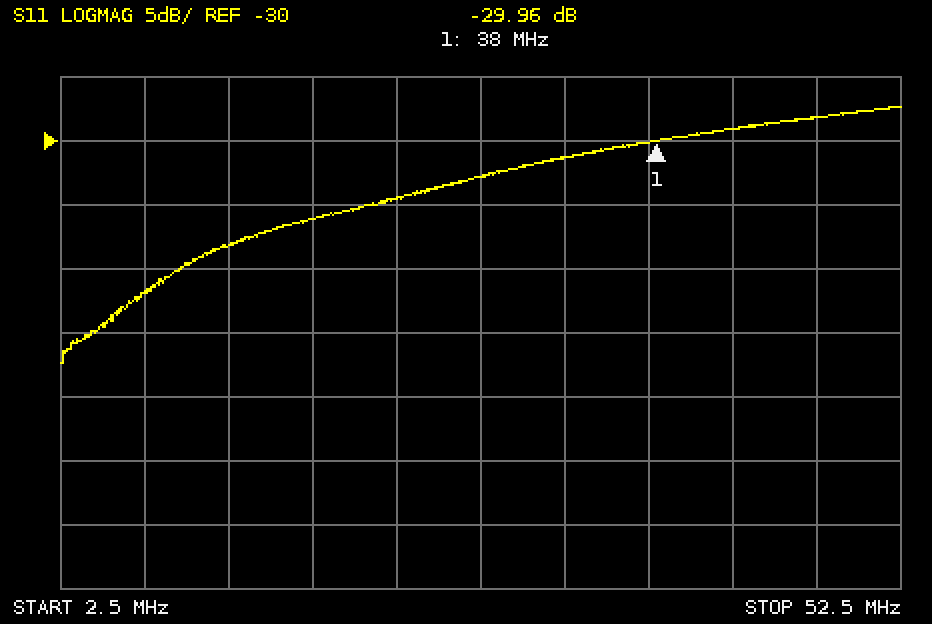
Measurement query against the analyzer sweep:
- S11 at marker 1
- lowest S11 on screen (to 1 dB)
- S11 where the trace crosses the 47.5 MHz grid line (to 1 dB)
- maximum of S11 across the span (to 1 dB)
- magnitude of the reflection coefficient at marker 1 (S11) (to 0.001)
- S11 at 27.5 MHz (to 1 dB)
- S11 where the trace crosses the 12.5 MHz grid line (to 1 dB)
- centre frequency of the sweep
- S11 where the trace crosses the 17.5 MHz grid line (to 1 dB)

-29.96 dB
-47 dB
-28 dB
-27 dB
0.032
-33 dB
-38 dB
27.5 MHz
-36 dB
